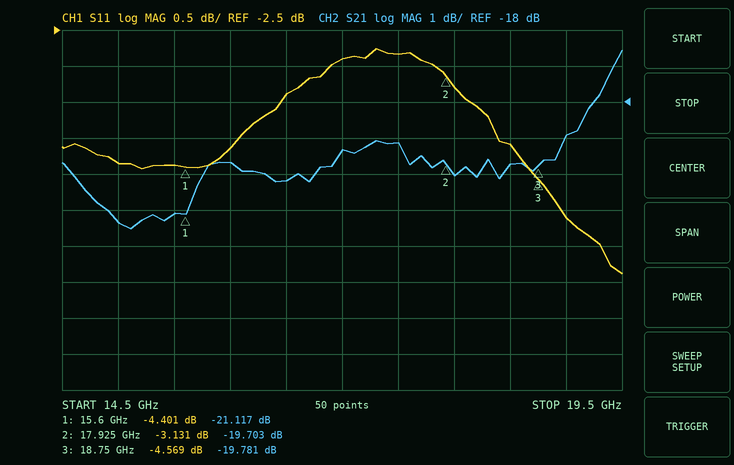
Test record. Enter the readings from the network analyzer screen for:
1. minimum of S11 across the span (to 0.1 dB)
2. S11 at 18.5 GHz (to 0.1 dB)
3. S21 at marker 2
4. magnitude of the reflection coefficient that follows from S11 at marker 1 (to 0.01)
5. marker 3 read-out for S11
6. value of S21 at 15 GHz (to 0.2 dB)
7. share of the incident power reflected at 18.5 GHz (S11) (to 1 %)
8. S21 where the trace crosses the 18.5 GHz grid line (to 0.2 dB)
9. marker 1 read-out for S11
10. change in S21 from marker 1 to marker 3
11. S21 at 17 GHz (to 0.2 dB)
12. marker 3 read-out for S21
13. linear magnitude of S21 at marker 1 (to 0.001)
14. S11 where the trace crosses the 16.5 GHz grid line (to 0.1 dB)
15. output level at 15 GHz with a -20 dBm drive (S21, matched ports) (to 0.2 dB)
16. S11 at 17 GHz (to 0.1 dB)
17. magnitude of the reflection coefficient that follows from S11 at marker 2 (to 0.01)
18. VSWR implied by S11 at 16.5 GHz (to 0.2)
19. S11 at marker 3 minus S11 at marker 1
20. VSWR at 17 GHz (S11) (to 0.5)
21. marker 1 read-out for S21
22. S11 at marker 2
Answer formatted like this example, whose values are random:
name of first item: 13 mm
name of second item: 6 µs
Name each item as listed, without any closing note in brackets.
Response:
minimum of S11 across the span: -5.9 dB
S11 at 18.5 GHz: -4.1 dB
S21 at marker 2: -19.703 dB
magnitude of the reflection coefficient that follows from S11 at marker 1: 0.60
marker 3 read-out for S11: -4.569 dB
value of S21 at 15 GHz: -21.4 dB
share of the incident power reflected at 18.5 GHz (S11): 39 %
S21 where the trace crosses the 18.5 GHz grid line: -19.8 dB
marker 1 read-out for S11: -4.401 dB
change in S21 from marker 1 to marker 3: 1.336 dB
S21 at 17 GHz: -19.4 dB
marker 3 read-out for S21: -19.781 dB
linear magnitude of S21 at marker 1: 0.088
S11 where the trace crosses the 16.5 GHz grid line: -3.4 dB
output level at 15 GHz with a -20 dBm drive (S21, matched ports): -41.4 dBm
S11 at 17 GHz: -2.9 dB
magnitude of the reflection coefficient that follows from S11 at marker 2: 0.70
VSWR implied by S11 at 16.5 GHz: 5.2
S11 at marker 3 minus S11 at marker 1: -0.168 dB
VSWR at 17 GHz (S11): 6.0
marker 1 read-out for S21: -21.117 dB
S11 at marker 2: -3.131 dB
